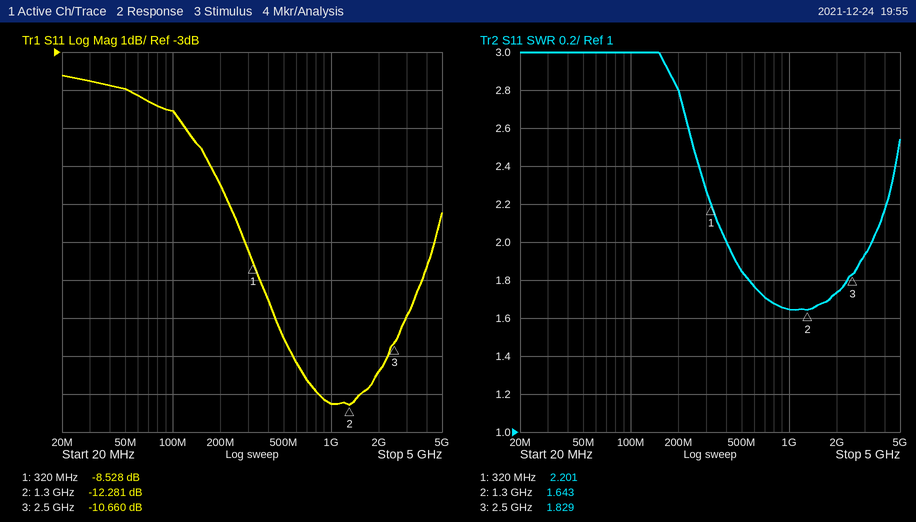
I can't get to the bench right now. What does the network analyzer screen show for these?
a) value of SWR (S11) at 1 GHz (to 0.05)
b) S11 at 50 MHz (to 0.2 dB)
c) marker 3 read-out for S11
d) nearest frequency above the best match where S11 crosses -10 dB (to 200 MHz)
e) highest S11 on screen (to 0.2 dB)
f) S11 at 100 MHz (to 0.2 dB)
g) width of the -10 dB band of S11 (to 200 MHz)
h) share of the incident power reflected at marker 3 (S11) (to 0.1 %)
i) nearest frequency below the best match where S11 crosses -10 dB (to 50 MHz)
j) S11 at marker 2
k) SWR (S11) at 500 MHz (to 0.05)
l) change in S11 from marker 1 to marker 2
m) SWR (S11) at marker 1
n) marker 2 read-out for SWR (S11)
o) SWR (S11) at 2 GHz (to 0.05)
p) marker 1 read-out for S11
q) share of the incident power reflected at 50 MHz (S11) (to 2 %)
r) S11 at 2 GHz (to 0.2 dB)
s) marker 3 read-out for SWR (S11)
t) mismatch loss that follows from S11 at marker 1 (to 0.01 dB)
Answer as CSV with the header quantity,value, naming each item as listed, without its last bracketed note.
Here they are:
quantity,value
value of SWR (S11) at 1 GHz,1.65
S11 at 50 MHz,-4.0 dB
marker 3 read-out for S11,-10.660 dB
nearest frequency above the best match where S11 crosses -10 dB,3.0 GHz
highest S11 on screen,-3.6 dB
S11 at 100 MHz,-4.6 dB
width of the -10 dB band of S11,2.6 GHz
share of the incident power reflected at marker 3 (S11),8.6 %
nearest frequency below the best match where S11 crosses -10 dB,450 MHz
S11 at marker 2,-12.281 dB
SWR (S11) at 500 MHz,1.85
change in S11 from marker 1 to marker 2,-3.753 dB
SWR (S11) at marker 1,2.201
marker 2 read-out for SWR,1.643
SWR (S11) at 2 GHz,1.75
marker 1 read-out for S11,-8.528 dB
share of the incident power reflected at 50 MHz (S11),40 %
S11 at 2 GHz,-11.4 dB
marker 3 read-out for SWR,1.829
mismatch loss that follows from S11 at marker 1,0.66 dB
